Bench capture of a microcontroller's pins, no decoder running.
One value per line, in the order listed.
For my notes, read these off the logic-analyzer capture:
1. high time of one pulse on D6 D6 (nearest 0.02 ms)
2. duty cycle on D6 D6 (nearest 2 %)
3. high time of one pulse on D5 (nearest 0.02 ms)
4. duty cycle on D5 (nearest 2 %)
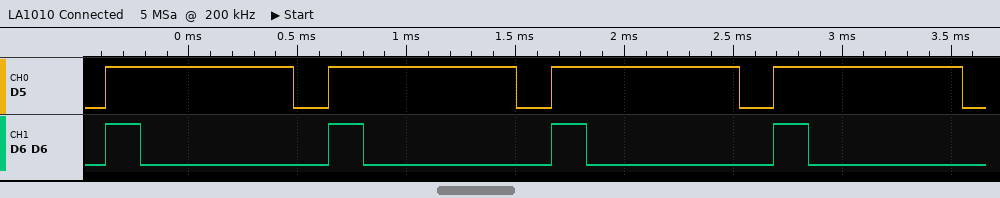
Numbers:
0.16 ms
16 %
0.86 ms
84 %
